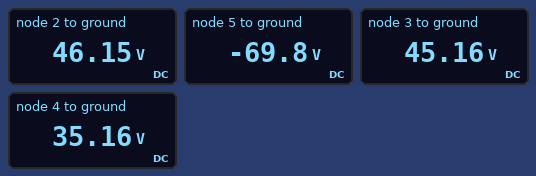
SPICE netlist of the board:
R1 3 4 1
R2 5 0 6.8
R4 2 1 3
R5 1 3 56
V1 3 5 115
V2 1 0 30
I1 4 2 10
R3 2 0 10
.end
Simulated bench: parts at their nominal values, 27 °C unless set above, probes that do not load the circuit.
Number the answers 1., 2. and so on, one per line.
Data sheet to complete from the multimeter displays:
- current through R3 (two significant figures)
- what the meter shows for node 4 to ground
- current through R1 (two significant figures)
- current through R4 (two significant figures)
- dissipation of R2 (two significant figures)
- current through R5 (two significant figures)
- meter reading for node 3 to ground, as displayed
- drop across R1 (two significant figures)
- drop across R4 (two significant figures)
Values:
1. 4.6 A
2. 35.16 V
3. 10 A
4. 5.4 A
5. 720 W
6. 270 mA
7. 45.16 V
8. 10 V
9. 16 V
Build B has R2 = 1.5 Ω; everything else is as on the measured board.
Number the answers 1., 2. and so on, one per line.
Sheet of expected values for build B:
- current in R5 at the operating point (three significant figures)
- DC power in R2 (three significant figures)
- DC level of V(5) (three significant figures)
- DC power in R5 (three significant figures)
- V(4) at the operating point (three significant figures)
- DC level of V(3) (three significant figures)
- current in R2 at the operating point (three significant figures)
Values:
1. 1.22 A
2. 189 W
3. -16.8 V
4. 83.0 W
5. 88.2 V
6. 98.2 V
7. 11.2 A
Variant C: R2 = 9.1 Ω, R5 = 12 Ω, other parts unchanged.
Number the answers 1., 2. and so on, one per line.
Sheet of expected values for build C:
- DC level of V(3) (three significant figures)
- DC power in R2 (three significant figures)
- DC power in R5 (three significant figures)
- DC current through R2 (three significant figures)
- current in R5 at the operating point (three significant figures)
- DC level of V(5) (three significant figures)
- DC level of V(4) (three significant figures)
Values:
1. 26.6 V
2. 859 W
3. 970 mW
4. 9.72 A
5. 284 mA
6. -88.4 V
7. 16.6 V
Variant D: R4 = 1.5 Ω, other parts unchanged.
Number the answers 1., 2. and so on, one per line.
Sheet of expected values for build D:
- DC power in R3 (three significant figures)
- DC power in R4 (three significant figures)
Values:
1. 153 W
2. 55.6 W
